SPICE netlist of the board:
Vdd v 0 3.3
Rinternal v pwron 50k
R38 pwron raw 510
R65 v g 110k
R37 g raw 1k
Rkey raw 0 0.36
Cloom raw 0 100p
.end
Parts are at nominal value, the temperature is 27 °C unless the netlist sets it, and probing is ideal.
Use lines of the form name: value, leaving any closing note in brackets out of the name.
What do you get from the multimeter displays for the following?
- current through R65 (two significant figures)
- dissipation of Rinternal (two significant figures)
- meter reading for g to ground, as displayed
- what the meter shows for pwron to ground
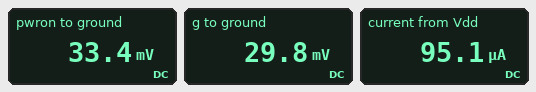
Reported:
current through R65: 30 µA
dissipation of Rinternal: 210 µW
meter reading for g to ground, as displayed: 29.8 mV
what the meter shows for pwron to ground: 33.4 mV
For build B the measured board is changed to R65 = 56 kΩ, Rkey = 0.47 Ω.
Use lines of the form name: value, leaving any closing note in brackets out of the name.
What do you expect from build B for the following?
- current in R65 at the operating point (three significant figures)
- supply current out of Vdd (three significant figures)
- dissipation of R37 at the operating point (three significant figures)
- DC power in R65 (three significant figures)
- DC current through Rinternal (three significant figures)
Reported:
current in R65 at the operating point: 57.9 µA
supply current out of Vdd: 123 µA
dissipation of R37 at the operating point: 3.35 µW
DC power in R65: 188 µW
DC current through Rinternal: 65.3 µA
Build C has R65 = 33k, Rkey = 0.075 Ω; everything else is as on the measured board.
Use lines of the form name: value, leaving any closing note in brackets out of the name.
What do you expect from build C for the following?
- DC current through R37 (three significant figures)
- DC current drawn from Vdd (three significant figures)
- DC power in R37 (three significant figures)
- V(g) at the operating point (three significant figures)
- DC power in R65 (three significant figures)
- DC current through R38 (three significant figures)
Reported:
DC current through R37: 97.1 µA
DC current drawn from Vdd: 162 µA
DC power in R37: 9.42 µW
V(g) at the operating point: 97.1 mV
DC power in R65: 311 µW
DC current through R38: 65.3 µA
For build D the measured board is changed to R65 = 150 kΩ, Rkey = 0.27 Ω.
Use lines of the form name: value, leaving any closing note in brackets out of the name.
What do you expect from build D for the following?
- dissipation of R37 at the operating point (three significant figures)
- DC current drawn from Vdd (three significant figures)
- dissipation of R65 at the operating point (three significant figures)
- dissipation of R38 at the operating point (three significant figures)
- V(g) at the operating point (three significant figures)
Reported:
dissipation of R37 at the operating point: 478 nW
DC current drawn from Vdd: 87.2 µA
dissipation of R65 at the operating point: 71.6 µW
dissipation of R38 at the operating point: 2.18 µW
V(g) at the operating point: 21.9 mV
